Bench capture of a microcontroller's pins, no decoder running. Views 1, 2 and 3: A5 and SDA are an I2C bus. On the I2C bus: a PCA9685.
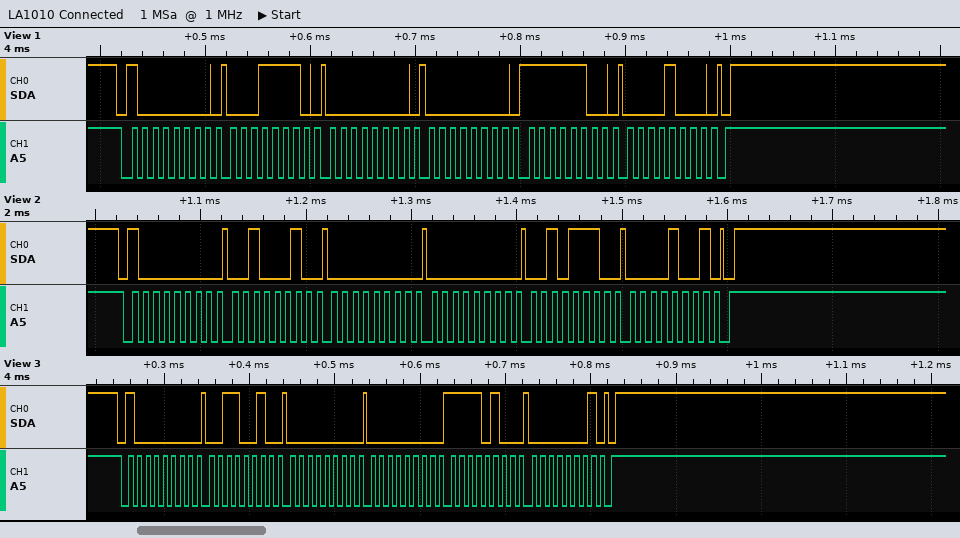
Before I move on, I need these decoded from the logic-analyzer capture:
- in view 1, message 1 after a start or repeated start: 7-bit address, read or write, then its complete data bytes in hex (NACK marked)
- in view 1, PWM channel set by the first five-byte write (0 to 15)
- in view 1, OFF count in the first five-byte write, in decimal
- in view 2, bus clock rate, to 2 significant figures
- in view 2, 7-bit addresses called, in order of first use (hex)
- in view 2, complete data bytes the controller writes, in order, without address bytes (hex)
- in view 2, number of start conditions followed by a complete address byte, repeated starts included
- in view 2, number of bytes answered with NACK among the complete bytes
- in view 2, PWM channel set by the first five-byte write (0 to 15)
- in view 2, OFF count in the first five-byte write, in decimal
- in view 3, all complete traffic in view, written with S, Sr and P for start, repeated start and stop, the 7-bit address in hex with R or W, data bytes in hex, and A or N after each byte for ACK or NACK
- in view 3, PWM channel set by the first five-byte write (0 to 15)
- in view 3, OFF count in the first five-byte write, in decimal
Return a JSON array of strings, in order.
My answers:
["0x40 write: 1E 00 00 FC 08", "6", "2300", "100 kHz", "0x40", "22 00 00 2E 09", "1", "0", "7", "2350", "S 40W A 32 A 00 A 00 A F4 A 01 A P", "11", "500"]
